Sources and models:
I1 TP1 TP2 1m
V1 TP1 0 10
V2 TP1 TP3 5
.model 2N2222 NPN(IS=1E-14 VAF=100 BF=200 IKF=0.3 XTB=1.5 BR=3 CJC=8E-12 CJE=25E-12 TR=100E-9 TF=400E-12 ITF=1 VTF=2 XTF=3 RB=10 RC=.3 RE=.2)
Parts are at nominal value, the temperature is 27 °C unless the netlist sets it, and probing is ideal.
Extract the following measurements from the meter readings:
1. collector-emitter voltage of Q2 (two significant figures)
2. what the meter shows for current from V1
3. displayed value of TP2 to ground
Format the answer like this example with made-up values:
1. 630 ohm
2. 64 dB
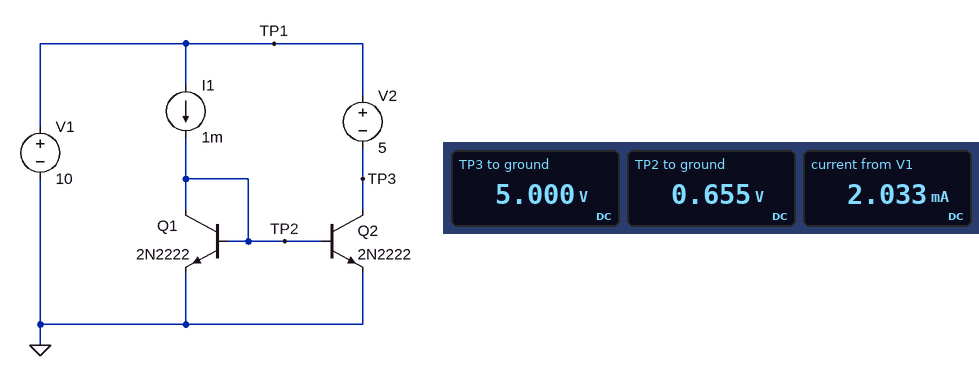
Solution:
1. 5.0 V
2. 2.033 mA
3. 0.655 V
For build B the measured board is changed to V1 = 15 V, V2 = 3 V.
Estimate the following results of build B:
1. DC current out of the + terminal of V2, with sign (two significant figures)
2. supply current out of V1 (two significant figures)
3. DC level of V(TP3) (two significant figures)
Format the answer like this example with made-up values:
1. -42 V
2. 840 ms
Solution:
1. -1.1 mA
2. 2.1 mA
3. 12 V
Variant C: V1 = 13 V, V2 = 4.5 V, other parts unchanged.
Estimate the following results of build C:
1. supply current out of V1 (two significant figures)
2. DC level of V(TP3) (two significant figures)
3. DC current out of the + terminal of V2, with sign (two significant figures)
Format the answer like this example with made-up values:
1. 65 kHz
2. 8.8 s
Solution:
1. 2.1 mA
2. 8.5 V
3. -1.1 mA
